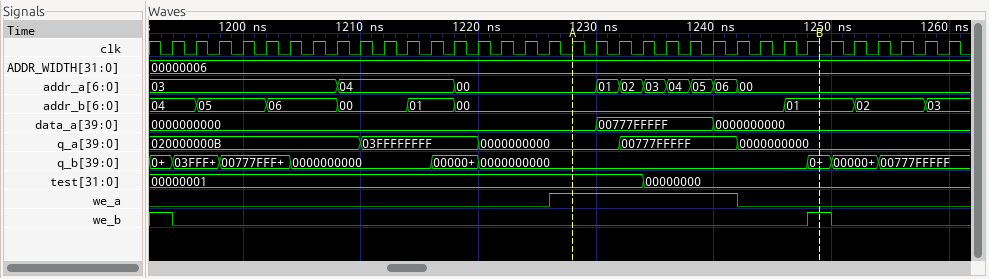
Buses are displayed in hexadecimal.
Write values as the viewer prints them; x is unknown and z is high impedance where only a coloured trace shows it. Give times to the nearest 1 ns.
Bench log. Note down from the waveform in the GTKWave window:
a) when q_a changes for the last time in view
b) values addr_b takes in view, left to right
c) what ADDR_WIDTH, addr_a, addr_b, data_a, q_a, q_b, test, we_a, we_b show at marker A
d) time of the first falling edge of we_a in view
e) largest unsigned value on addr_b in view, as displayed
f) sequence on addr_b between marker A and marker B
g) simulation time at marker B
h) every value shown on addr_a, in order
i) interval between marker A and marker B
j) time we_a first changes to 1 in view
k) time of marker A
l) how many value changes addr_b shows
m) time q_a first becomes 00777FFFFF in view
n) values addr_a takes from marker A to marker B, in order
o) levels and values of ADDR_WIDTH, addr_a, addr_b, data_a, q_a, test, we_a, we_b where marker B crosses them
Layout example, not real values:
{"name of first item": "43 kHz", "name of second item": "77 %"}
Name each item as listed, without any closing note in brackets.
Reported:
{"when q_a changes for the last time in view": "1242 ns", "values addr_b takes in view, left to right": "04, 05, 06, 00, 01, 00, 01, 02, 03", "what ADDR_WIDTH, addr_a, addr_b, data_a, q_a, q_b, test, we_a, we_b show at marker A": "ADDR_WIDTH=00000006, addr_a=00, addr_b=00, data_a=0000000000, q_a=0000000000, q_b=0000000000, test=00000001, we_a=1, we_b=0", "time of the first falling edge of we_a in view": "1242 ns", "largest unsigned value on addr_b in view, as displayed": "06", "sequence on addr_b between marker A and marker B": "00, 01", "simulation time at marker B": "1249 ns", "every value shown on addr_a, in order": "03, 04, 00, 01, 02, 03, 04, 05, 06, 00", "interval between marker A and marker B": "21 ns", "time we_a first changes to 1 in view": "1226 ns", "time of marker A": "1228 ns", "how many value changes addr_b shows": "8", "time q_a first becomes 00777FFFFF in view": "1232 ns", "values addr_a takes from marker A to marker B, in order": "00, 01, 02, 03, 04, 05, 06, 00", "levels and values of ADDR_WIDTH, addr_a, addr_b, data_a, q_a, test, we_a, we_b where marker B crosses them": "ADDR_WIDTH=00000006, addr_a=00, addr_b=01, data_a=0000000000, q_a=0000000000, test=00000000, we_a=0, we_b=1"}
